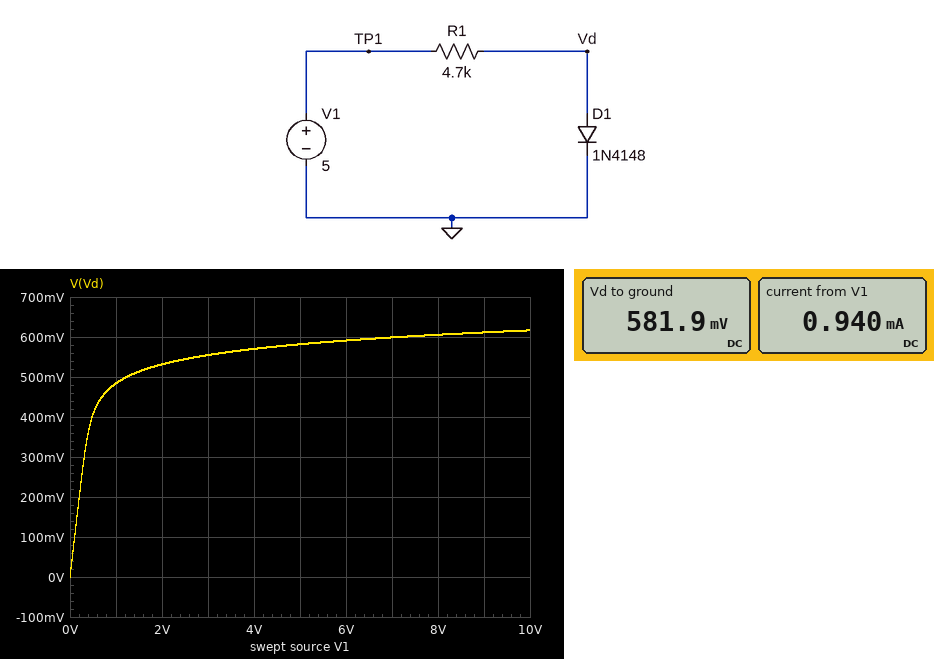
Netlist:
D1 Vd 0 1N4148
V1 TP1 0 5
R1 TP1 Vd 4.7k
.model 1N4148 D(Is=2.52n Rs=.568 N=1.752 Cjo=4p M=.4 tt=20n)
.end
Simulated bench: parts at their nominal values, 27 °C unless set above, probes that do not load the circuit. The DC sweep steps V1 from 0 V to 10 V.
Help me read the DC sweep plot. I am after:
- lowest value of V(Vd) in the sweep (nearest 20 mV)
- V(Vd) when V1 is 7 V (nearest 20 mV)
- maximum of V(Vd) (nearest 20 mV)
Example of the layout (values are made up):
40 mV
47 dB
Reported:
0 V
600 mV
620 mV
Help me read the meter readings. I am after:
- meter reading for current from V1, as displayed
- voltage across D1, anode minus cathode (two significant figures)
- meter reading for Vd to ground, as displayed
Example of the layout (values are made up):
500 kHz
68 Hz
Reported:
0.940 mA
580 mV
581.9 mV
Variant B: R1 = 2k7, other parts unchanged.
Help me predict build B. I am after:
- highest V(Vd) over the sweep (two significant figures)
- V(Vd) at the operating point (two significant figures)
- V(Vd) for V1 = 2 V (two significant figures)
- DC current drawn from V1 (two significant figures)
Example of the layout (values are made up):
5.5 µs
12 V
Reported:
640 mV
610 mV
560 mV
1.6 mA
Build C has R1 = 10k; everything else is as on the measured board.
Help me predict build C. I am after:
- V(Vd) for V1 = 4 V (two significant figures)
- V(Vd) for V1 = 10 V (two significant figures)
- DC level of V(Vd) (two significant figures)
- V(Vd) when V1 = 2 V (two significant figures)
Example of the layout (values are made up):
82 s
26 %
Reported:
540 mV
580 mV
550 mV
500 mV
